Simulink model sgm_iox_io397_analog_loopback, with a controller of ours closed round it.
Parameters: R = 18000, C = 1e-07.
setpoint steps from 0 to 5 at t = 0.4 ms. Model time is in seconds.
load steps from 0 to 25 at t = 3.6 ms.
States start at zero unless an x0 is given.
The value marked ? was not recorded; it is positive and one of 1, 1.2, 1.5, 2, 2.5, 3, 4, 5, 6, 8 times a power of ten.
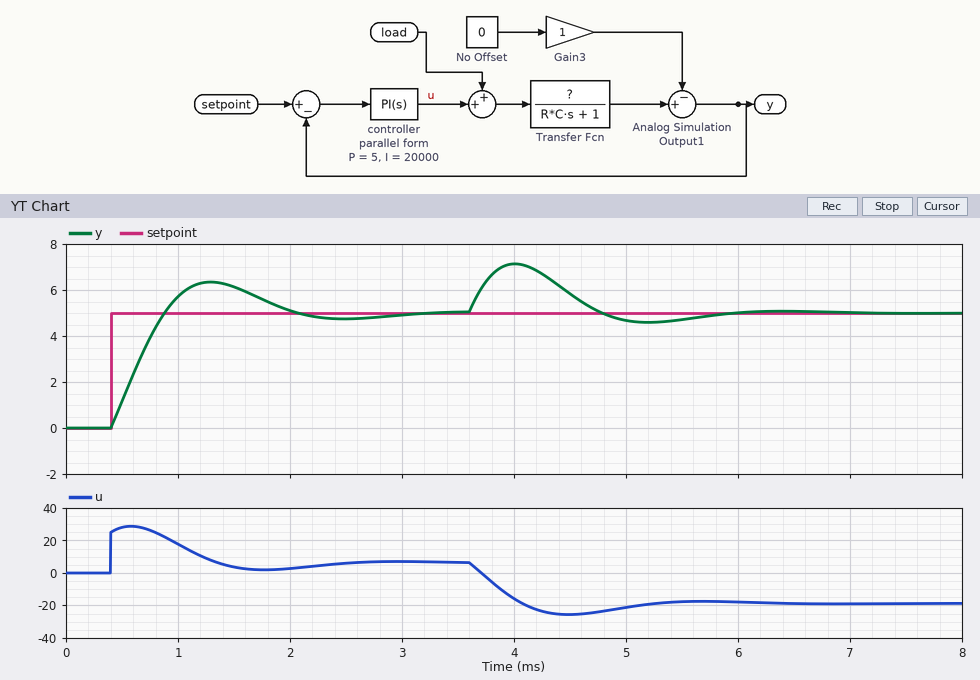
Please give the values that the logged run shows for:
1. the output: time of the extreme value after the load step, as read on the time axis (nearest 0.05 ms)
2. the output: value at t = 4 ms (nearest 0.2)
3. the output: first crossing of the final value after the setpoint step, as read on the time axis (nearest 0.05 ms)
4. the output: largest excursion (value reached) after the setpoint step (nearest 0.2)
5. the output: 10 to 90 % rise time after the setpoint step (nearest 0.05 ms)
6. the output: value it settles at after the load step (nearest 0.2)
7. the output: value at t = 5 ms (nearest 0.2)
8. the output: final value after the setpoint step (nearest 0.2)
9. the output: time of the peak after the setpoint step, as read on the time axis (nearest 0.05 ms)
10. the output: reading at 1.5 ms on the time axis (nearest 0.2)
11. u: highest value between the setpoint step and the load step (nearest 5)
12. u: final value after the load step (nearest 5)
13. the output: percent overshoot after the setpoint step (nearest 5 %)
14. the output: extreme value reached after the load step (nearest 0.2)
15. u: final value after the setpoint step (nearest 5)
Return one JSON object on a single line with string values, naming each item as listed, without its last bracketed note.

{"the output: time of the extreme value after the load step, as read on the time axis": "4.00 ms", "the output: value at t = 4 ms": "7.2", "the output: first crossing of the final value after the setpoint step, as read on the time axis": "0.90 ms", "the output: largest excursion (value reached) after the setpoint step": "6.4", "the output: 10 to 90 % rise time after the setpoint step": "0.35 ms", "the output: value it settles at after the load step": "5.0", "the output: value at t = 5 ms": "4.6", "the output: final value after the setpoint step": "5.0", "the output: time of the peak after the setpoint step, as read on the time axis": "1.30 ms", "the output: reading at 1.5 ms on the time axis": "6.2", "u: highest value between the setpoint step and the load step": "30", "u: final value after the load step": "-20", "the output: percent overshoot after the setpoint step": "25 %", "the output: extreme value reached after the load step": "7.2", "u: final value after the setpoint step": "5"}
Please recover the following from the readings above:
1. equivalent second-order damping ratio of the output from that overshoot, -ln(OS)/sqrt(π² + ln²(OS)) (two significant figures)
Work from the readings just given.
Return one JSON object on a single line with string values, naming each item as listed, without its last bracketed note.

{"equivalent second-order damping ratio of the output from that overshoot, -ln(OS)/sqrt(π² + ln²(OS))": "0.40"}
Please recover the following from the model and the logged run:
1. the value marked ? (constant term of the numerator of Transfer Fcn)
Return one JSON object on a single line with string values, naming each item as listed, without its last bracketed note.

{"the value marked ?": "0.8"}
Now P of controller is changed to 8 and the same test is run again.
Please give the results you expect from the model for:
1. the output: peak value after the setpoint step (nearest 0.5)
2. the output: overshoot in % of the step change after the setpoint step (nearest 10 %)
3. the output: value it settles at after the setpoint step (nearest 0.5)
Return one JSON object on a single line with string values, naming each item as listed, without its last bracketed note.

{"the output: peak value after the setpoint step": "6.0", "the output: overshoot in % of the step change after the setpoint step": "20 %", "the output: value it settles at after the setpoint step": "5.0"}
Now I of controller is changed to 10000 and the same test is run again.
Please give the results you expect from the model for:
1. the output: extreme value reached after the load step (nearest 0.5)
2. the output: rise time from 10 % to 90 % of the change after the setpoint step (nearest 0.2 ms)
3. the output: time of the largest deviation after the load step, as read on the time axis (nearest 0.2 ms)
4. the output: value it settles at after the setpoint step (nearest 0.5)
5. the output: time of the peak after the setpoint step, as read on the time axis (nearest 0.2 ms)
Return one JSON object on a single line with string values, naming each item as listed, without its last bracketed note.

{"the output: extreme value reached after the load step": "7.5", "the output: rise time from 10 % to 90 % of the change after the setpoint step": "0.6 ms", "the output: time of the largest deviation after the load step, as read on the time axis": "4.2 ms", "the output: value it settles at after the setpoint step": "5.0", "the output: time of the peak after the setpoint step, as read on the time axis": "1.6 ms"}
